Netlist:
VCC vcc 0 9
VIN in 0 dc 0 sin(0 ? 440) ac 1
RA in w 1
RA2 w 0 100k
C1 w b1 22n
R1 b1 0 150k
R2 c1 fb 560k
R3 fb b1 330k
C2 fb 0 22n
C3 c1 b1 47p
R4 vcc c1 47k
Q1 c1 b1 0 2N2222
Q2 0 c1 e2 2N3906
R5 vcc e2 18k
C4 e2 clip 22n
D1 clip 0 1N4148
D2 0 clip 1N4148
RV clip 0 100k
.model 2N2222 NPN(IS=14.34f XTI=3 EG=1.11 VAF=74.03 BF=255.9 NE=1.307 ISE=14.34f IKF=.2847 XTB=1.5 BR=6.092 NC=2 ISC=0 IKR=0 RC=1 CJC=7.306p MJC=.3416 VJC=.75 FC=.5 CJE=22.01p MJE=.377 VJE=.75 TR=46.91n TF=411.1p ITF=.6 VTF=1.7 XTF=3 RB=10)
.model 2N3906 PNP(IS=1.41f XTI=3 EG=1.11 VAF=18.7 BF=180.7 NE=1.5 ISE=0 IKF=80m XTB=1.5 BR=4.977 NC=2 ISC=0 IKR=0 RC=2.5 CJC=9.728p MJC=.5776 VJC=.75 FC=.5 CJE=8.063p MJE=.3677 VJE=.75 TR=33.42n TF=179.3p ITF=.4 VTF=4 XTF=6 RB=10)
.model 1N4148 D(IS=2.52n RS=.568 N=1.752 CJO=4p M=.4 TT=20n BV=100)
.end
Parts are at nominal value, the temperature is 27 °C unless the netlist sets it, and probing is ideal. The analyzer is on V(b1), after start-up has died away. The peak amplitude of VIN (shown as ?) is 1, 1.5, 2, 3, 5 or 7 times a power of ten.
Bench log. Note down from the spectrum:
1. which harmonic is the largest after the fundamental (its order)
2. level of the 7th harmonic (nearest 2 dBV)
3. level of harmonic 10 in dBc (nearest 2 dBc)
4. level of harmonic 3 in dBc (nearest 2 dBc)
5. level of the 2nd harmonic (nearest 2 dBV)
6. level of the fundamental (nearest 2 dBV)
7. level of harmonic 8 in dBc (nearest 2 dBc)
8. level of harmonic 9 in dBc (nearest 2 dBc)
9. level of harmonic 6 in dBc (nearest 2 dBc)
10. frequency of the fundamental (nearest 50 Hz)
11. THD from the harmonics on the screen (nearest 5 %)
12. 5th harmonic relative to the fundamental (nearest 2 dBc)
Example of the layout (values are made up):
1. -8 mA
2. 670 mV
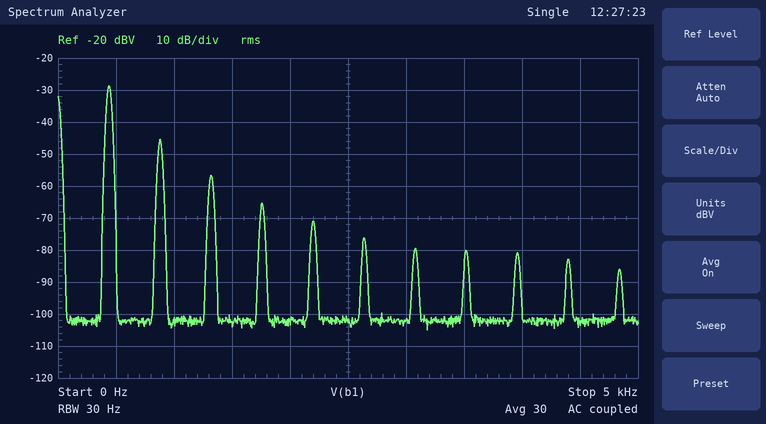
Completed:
1. 2
2. -80 dBV
3. -54 dBc
4. -28 dBc
5. -46 dBV
6. -28 dBV
7. -52 dBc
8. -52 dBc
9. -48 dBc
10. 450 Hz
11. 15 %
12. -42 dBc
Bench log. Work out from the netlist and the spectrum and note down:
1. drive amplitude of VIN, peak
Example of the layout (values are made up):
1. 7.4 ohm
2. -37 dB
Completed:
1. 70 mV
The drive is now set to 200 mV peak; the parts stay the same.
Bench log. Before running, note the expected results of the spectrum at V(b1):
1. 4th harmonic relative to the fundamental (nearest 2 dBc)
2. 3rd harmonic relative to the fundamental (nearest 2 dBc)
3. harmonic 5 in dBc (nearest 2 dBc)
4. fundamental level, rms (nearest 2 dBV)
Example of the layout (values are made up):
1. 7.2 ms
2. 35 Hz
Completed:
1. -34 dBc
2. -24 dBc
3. -38 dBc
4. -20 dBV
